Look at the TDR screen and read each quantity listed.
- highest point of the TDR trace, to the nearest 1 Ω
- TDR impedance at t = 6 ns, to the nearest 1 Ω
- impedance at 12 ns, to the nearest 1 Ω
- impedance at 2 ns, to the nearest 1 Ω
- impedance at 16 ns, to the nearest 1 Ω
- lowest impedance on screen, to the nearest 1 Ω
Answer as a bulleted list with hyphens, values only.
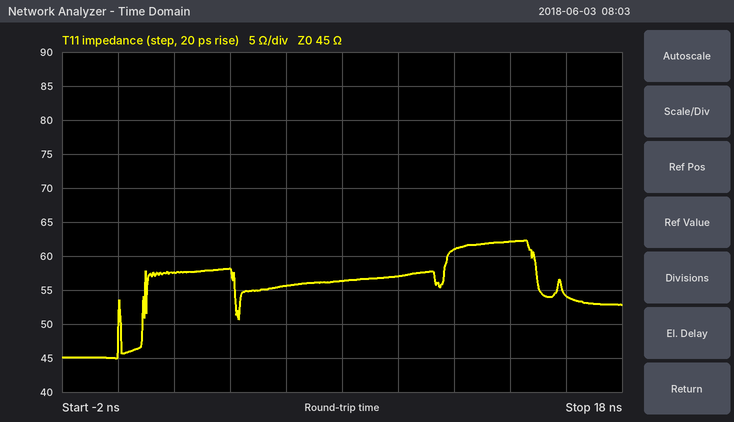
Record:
- 62 Ω
- 56 Ω
- 61 Ω
- 58 Ω
- 54 Ω
- 45 Ω
